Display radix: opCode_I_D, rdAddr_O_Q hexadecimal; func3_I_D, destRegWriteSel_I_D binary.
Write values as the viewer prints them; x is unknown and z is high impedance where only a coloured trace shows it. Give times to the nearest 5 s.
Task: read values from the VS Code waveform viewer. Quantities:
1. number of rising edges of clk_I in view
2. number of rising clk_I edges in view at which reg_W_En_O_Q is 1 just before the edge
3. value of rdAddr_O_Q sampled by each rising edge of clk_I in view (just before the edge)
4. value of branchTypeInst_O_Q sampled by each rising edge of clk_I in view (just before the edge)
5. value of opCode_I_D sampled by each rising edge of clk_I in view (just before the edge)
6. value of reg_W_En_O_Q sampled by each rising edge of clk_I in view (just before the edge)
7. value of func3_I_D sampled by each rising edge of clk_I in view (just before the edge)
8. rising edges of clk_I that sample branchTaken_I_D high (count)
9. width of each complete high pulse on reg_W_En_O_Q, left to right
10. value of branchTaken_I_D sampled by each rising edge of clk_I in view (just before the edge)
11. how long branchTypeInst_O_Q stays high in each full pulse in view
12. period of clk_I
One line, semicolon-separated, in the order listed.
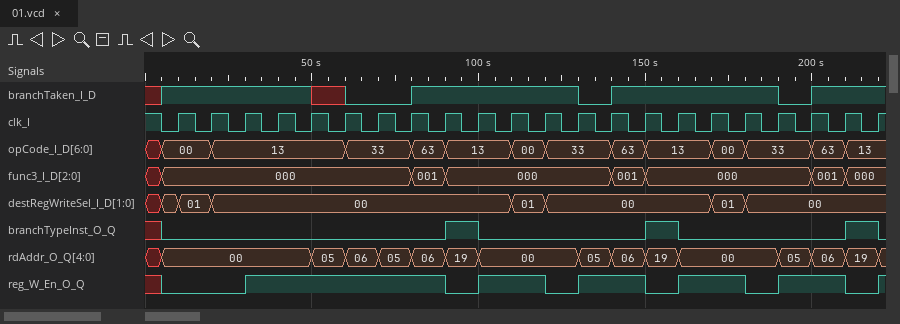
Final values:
22; 14; 00, 00, 00, 00, 00, 05, 06, 05, 06, 19, 00, 00, 00, 05, 06, 19, 00, 00, 00, 05, 06, 19; 0 0 0 0 0 0 0 0 0 1 0 0 0 0 0 1 0 0 0 0 0 1; 00, 00, 13, 13, 13, 13, 33, 33, 63, 13, 13, 00, 33, 33, 63, 13, 13, 00, 33, 33, 63, 13; 0 0 0 1 1 1 1 1 1 0 1 1 0 1 1 0 1 1 0 1 1 0; 000, 000, 000, 000, 000, 000, 000, 000, 001, 000, 000, 000, 000, 000, 001, 000, 000, 000, 000, 000, 001, 000; 17; 60 s, 20 s, 20 s, 20 s, 20 s; 1 1 1 1 1 x 0 0 1 1 1 1 1 0 1 1 1 1 1 0 1 1; 10 s, 10 s, 10 s; 10 s
